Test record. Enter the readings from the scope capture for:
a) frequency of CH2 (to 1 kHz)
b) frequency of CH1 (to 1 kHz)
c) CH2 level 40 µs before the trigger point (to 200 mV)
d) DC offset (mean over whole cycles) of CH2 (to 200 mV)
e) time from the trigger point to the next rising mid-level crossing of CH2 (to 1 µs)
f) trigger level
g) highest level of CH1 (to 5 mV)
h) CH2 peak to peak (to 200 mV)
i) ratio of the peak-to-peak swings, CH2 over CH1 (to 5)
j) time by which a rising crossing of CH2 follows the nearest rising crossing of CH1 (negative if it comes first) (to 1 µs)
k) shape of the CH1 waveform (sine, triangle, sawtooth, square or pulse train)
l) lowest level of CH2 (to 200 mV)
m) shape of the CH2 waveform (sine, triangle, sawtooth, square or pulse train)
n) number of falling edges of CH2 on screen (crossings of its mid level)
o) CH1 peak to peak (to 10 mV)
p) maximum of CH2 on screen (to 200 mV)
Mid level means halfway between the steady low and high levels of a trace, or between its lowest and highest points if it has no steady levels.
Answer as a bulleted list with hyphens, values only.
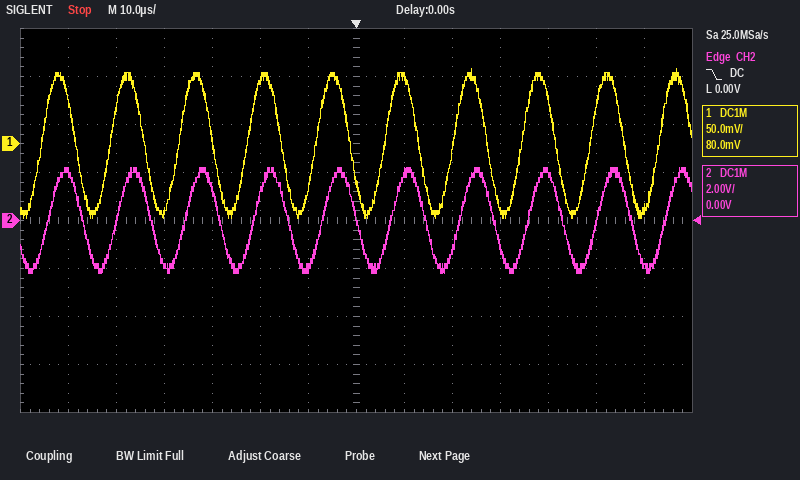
- 70 kHz
- 70 kHz
- -1.8 V
- 0.0 V
- 7 µs
- 0.00 V
- 80 mV
- 4.4 V
- 30
- +1 µs
- sine
- -2.2 V
- sine
- 9
- 160 mV
- 2.2 V
